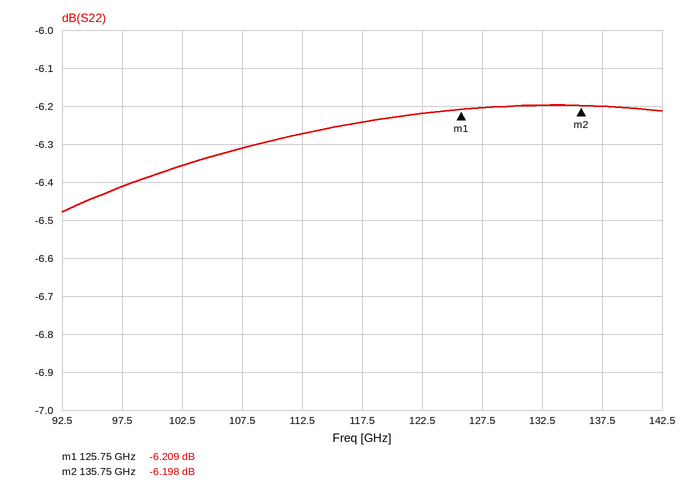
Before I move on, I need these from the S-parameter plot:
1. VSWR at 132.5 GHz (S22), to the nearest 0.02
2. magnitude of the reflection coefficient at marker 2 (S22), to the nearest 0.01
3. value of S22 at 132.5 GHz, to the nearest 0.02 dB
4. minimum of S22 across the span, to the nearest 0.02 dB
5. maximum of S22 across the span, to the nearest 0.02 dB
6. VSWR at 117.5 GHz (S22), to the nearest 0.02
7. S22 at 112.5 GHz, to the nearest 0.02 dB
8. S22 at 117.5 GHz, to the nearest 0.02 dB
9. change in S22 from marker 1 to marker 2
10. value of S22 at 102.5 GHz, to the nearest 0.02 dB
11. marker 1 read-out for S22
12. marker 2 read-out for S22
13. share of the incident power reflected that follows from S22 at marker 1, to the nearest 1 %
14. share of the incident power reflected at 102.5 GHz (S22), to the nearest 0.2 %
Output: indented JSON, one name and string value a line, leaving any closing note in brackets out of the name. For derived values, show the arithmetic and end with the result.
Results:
{
  "VSWR at 132.5 GHz (S22), to the nearest 0.02": "|Γ| = 10^(-6.2/20) = 0.4898; VSWR = (1 + 0.4898)/(1 − 0.4898) ≈ 2.92",
  "magnitude of the reflection coefficient at marker 2 (S22), to the nearest 0.01": "10^(-6.198/20) ≈ 0.49",
  "value of S22 at 132.5 GHz, to the nearest 0.02 dB": "-6.20 dB",
  "minimum of S22 across the span, to the nearest 0.02 dB": "-6.48 dB",
  "maximum of S22 across the span, to the nearest 0.02 dB": "-6.20 dB",
  "VSWR at 117.5 GHz (S22), to the nearest 0.02": "|Γ| = 10^(-6.24/20) = 0.4875; VSWR = (1 + 0.4875)/(1 − 0.4875) ≈ 2.90",
  "S22 at 112.5 GHz, to the nearest 0.02 dB": "-6.28 dB",
  "S22 at 117.5 GHz, to the nearest 0.02 dB": "-6.24 dB",
  "change in S22 from marker 1 to marker 2": "-6.198 − (-6.209) = 0.011 dB",
  "value of S22 at 102.5 GHz, to the nearest 0.02 dB": "-6.36 dB",
  "marker 1 read-out for S22": "-6.209 dB",
  "marker 2 read-out for S22": "-6.198 dB",
  "share of the incident power reflected that follows from S22 at marker 1, to the nearest 1 %": "10^(-6.209/10) ≈ 24 %",
  "share of the incident power reflected at 102.5 GHz (S22), to the nearest 0.2 %": "10^(-6.36/10) ≈ 23.1 %, so 23.2 % to the nearest 0.2 %"
}
